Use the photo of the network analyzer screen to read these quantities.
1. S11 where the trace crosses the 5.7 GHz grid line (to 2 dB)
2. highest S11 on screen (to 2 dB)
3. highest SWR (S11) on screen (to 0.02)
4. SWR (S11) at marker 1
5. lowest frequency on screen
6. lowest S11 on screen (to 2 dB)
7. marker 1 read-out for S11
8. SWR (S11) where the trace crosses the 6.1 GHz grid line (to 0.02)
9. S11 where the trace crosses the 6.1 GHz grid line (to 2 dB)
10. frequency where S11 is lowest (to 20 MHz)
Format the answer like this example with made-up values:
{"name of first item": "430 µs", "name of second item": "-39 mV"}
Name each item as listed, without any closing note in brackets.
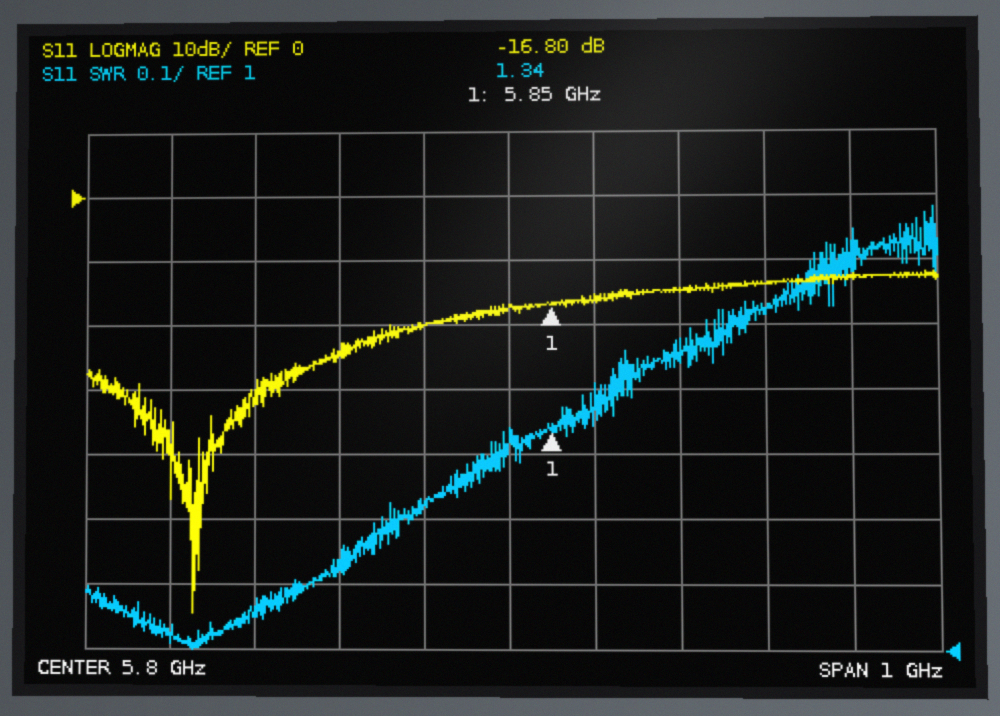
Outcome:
{"S11 where the trace crosses the 5.7 GHz grid line": "-20 dB", "highest S11 on screen": "-12 dB", "highest SWR (S11) on screen": "1.68", "SWR (S11) at marker 1": "1.34", "lowest frequency on screen": "5.3 GHz", "lowest S11 on screen": "-64 dB", "marker 1 read-out for S11": "-16.80 dB", "SWR (S11) where the trace crosses the 6.1 GHz grid line": "1.52", "S11 where the trace crosses the 6.1 GHz grid line": "-14 dB", "frequency where S11 is lowest": "5.42 GHz"}
